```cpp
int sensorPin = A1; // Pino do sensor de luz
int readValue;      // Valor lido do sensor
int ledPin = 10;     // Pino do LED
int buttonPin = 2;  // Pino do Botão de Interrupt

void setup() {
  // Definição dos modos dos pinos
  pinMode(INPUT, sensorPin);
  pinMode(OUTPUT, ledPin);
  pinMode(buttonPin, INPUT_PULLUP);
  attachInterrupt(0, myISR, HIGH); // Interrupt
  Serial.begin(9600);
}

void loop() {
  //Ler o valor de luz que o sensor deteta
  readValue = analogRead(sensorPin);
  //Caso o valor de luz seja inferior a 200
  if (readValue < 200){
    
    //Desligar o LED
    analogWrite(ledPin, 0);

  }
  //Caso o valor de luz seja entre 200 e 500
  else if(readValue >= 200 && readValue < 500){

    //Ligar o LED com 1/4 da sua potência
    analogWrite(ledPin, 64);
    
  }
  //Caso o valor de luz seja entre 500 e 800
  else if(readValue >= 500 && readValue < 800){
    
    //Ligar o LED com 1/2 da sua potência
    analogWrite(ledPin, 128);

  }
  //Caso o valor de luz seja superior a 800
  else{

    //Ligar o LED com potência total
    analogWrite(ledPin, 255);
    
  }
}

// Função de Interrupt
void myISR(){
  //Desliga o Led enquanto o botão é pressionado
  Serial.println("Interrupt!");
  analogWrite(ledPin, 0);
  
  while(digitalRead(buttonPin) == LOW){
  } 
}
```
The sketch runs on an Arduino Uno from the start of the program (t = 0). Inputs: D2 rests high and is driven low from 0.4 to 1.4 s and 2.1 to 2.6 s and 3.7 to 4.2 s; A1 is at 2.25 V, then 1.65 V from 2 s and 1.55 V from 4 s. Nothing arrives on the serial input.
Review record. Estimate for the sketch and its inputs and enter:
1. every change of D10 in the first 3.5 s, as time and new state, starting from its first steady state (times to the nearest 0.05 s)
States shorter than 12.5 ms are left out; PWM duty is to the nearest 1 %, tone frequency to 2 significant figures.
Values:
0 s PWM 25 %; 0.4 s low; 1.4 s PWM 25 %; 2.1 s low; 2.6 s PWM 25 %
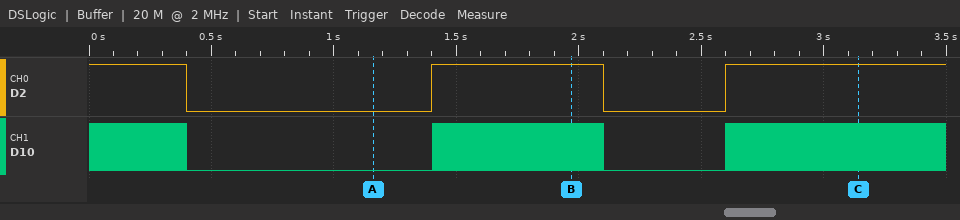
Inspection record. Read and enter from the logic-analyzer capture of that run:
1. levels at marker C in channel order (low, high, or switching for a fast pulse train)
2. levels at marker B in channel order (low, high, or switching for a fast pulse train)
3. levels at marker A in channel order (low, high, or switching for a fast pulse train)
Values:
D2 high, D10 switching
D2 high, D10 switching
D2 low, D10 low
